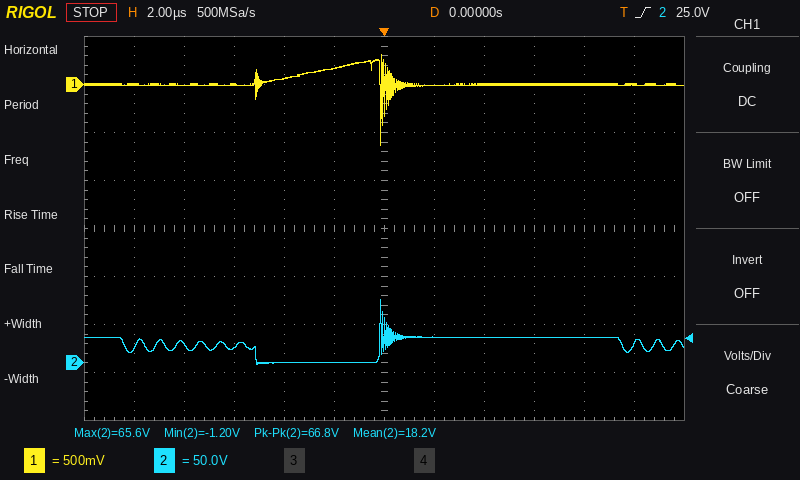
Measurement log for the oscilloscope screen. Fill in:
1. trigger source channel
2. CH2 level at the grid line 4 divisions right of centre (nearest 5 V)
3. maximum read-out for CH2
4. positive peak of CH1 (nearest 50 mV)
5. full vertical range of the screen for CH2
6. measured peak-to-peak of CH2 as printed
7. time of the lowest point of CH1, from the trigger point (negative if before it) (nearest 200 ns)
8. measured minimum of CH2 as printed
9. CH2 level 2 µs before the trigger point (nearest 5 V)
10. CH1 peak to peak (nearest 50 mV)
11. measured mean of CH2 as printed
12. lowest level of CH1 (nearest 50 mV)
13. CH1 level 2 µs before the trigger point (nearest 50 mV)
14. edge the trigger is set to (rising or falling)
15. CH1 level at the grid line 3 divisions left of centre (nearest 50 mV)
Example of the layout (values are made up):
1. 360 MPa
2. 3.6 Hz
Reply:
1. CH2
2. 25 V
3. 65.6 V
4. 300 mV
5. 400 V
6. 66.8 V
7. -200 ns
8. -1.20 V
9. 0 V
10. 950 mV
11. 18.2 V
12. -650 mV
13. 150 mV
14. rising
15. 0 mV
